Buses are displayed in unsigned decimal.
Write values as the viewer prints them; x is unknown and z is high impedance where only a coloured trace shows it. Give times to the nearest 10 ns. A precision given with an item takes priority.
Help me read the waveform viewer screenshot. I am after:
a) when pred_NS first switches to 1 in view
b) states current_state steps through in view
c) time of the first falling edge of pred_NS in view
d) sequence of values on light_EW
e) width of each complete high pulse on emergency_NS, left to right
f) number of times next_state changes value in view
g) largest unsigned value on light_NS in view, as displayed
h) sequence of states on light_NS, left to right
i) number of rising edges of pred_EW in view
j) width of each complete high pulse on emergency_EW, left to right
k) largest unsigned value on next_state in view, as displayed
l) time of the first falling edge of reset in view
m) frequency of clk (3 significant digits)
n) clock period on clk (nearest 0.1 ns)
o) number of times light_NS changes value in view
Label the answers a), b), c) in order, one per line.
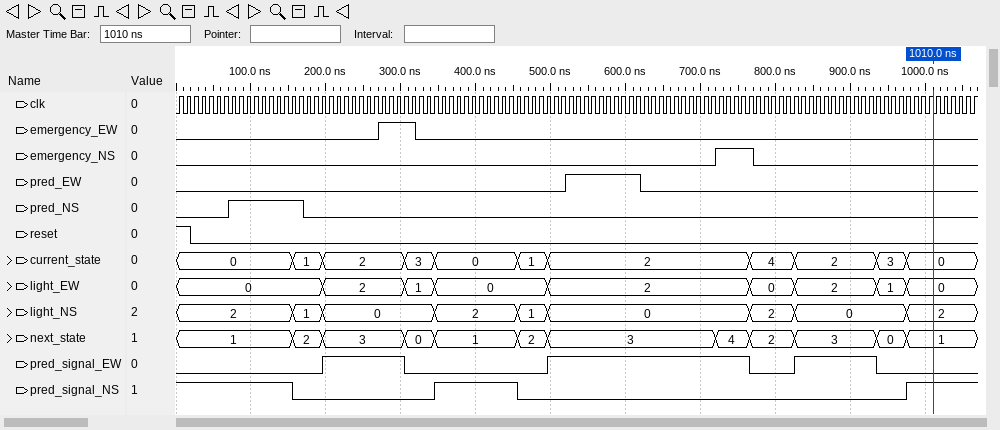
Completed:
a) 70 ns
b) 0, 1, 2, 3, 0, 1, 2, 4, 2, 3, 0
c) 170 ns
d) 0, 2, 1, 0, 2, 0, 2, 1, 0
e) 50 ns
f) 11
g) 2
h) 2, 1, 0, 2, 1, 0, 2, 0, 2
i) 1
j) 50 ns
k) 4
l) 20 ns
m) 100 MHz
n) 10 ns
o) 8
